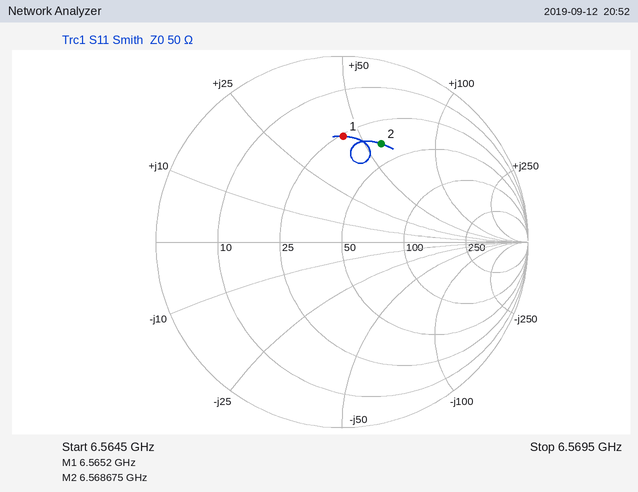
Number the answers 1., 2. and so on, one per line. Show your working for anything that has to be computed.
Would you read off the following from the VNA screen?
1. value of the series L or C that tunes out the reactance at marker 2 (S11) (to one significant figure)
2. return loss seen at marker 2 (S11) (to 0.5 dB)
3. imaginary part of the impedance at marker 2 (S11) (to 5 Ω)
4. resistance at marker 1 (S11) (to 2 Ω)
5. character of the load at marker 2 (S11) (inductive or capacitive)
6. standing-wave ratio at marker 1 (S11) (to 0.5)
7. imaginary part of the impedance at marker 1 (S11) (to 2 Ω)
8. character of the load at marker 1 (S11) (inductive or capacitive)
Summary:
1. C = 1/(2π × 6.568675 GHz × 60 Ω) ≈ 404 fF, so 400 fF to one significant figure
2. 5.0 dB
3. +60 Ω
4. 26 Ω
5. inductive
6. 3.5
7. +44 Ω
8. inductive
